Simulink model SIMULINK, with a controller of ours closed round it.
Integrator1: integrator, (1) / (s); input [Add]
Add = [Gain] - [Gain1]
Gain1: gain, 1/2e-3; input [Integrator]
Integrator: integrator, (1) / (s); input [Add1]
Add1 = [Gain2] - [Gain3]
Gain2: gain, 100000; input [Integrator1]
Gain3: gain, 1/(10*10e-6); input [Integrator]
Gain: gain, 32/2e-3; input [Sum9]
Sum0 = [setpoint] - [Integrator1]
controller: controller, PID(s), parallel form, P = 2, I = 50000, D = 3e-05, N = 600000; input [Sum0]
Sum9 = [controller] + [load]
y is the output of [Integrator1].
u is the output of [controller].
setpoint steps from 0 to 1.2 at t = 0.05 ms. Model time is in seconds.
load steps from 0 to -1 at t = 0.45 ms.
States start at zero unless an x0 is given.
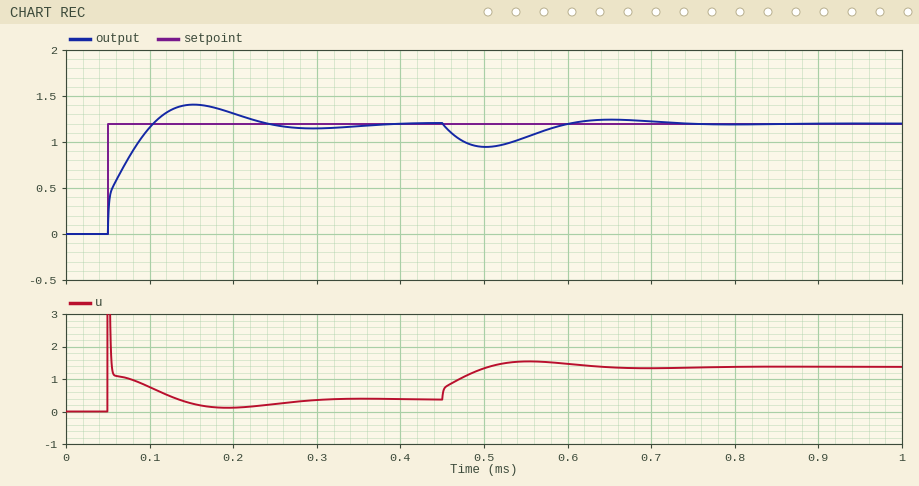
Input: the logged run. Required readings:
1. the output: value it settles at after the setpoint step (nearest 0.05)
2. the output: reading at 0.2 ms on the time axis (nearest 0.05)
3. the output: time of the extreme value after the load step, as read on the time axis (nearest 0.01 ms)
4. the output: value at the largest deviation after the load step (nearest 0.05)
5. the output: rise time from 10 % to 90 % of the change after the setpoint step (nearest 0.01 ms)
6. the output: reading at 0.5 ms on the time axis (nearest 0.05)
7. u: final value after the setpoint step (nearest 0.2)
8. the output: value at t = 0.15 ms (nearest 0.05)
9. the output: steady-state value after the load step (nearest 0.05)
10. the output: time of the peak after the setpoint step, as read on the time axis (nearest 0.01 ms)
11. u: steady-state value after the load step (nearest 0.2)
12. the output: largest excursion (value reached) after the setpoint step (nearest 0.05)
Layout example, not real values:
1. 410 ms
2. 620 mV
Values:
1. 1.20
2. 1.30
3. 0.50 ms
4. 0.95
5. 0.04 ms
6. 0.95
7. 0.4
8. 1.40
9. 1.20
10. 0.15 ms
11. 1.4
12. 1.40
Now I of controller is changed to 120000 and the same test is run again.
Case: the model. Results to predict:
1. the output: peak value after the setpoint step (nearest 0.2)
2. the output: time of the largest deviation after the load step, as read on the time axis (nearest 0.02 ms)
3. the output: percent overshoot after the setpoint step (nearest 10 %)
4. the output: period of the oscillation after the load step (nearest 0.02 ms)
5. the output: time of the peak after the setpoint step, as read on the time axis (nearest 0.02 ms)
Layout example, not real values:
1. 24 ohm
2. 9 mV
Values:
1. 1.6
2. 0.48 ms
3. 30 %
4. 0.18 ms
5. 0.12 ms
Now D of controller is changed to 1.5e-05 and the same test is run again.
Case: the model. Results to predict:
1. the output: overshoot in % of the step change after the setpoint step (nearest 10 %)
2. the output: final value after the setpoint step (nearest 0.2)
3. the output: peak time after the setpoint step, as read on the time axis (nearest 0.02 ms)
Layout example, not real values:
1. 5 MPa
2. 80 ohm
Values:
1. 20 %
2. 1.2
3. 0.14 ms
